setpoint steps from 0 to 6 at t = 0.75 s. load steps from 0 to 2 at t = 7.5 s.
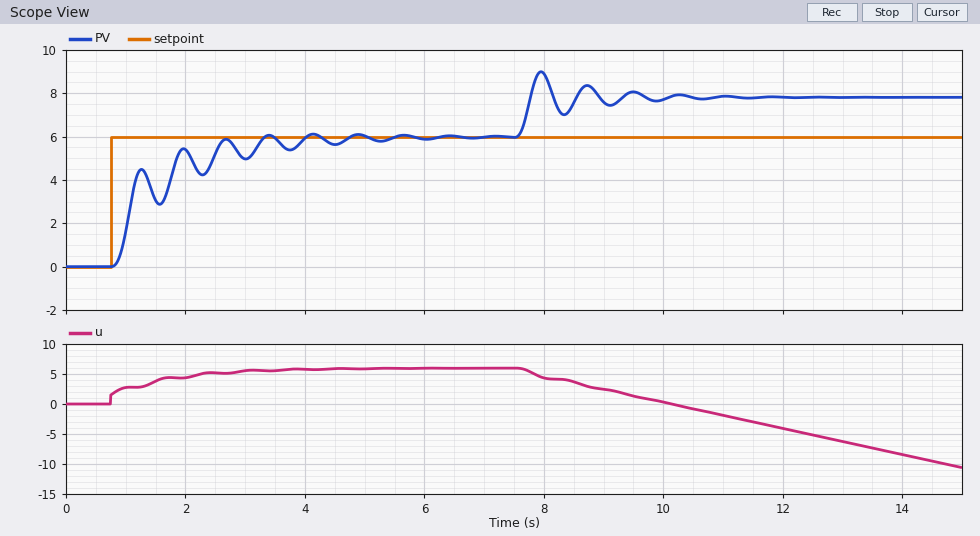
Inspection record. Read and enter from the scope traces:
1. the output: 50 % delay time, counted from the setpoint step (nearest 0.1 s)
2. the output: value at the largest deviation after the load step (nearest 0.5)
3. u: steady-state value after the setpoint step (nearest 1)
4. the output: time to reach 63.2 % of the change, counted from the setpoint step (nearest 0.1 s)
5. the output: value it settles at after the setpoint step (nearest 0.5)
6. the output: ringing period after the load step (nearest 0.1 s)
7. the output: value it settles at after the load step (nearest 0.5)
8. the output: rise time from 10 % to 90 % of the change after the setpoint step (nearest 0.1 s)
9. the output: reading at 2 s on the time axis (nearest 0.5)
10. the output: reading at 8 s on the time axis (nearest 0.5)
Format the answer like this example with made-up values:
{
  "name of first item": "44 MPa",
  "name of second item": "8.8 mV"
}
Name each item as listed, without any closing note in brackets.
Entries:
{
  "the output: 50 % delay time, counted from the setpoint step": "0.3 s",
  "the output: value at the largest deviation after the load step": "9.0",
  "u: steady-state value after the setpoint step": "6",
  "the output: time to reach 63.2 % of the change, counted from the setpoint step": "0.4 s",
  "the output: value it settles at after the setpoint step": "6.0",
  "the output: ringing period after the load step": "0.8 s",
  "the output: value it settles at after the load step": "8.0",
  "the output: rise time from 10 % to 90 % of the change after the setpoint step": "1.0 s",
  "the output: reading at 2 s on the time axis": "5.5",
  "the output: reading at 8 s on the time axis": "9.0"
}
